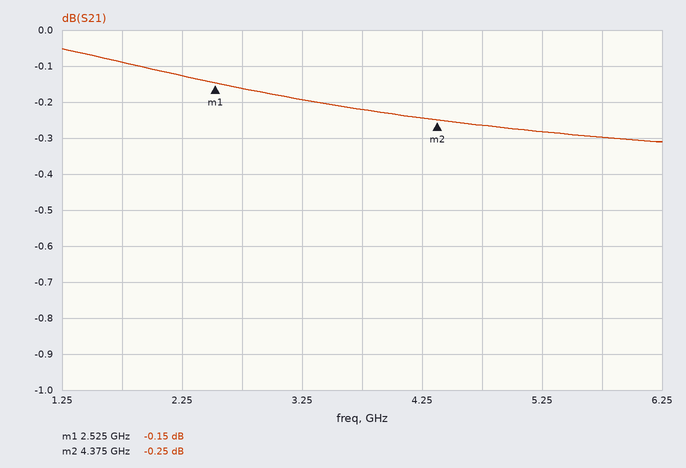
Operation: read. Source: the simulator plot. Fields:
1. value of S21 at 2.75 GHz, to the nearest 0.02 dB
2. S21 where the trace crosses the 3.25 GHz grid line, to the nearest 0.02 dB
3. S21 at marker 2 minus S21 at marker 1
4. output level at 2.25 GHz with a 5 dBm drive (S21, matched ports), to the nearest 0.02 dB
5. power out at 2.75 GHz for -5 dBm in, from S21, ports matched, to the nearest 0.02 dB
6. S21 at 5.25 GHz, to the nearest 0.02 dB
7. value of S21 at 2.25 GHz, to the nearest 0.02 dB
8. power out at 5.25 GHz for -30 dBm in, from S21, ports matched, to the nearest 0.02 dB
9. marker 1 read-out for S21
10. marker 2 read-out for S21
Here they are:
-0.16 dB
-0.20 dB
-0.10 dB
4.88 dBm
-5.16 dBm
-0.28 dB
-0.12 dB
-30.28 dBm
-0.15 dB
-0.25 dB
